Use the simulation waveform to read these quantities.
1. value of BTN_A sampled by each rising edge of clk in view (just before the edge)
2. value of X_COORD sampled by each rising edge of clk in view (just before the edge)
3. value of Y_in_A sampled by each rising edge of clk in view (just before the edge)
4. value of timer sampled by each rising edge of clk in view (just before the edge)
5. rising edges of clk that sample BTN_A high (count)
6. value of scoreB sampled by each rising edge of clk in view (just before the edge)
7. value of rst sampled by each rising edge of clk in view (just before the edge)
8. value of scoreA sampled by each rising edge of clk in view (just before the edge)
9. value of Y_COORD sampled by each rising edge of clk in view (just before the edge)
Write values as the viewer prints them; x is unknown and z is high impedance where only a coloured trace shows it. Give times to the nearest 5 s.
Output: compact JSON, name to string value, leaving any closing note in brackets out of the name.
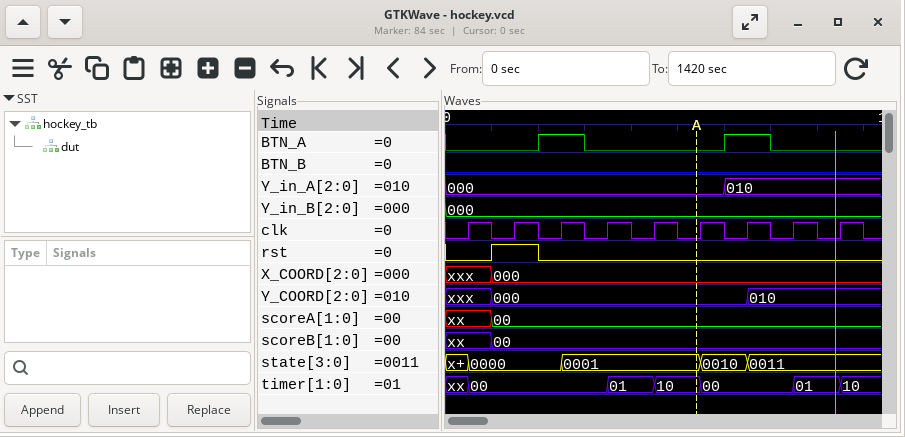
{"value of BTN_A sampled by each rising edge of clk in view": "0 0 1 0 0 0 1 0 0", "value of X_COORD sampled by each rising edge of clk in view": "xxx, 000, 000, 000, 000, 000, 000, 000, 000", "value of Y_in_A sampled by each rising edge of clk in view": "000, 000, 000, 000, 000, 000, 010, 010, 010", "value of timer sampled by each rising edge of clk in view": "xx, 00, 00, 00, 01, 10, 00, 00, 01", "rising edges of clk that sample BTN_A high": "2", "value of scoreB sampled by each rising edge of clk in view": "xx, 00, 00, 00, 00, 00, 00, 00, 00", "value of rst sampled by each rising edge of clk in view": "0 1 0 0 0 0 0 0 0", "value of scoreA sampled by each rising edge of clk in view": "xx, 00, 00, 00, 00, 00, 00, 00, 00", "value of Y_COORD sampled by each rising edge of clk in view": "xxx, 000, 000, 000, 000, 000, 000, 010, 010"}
